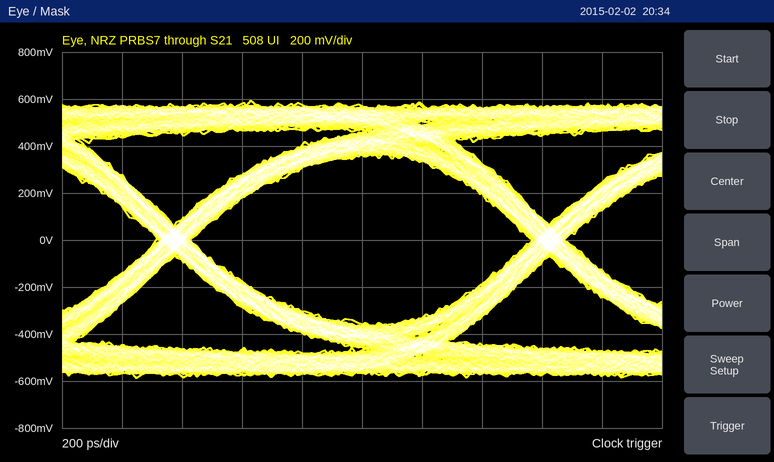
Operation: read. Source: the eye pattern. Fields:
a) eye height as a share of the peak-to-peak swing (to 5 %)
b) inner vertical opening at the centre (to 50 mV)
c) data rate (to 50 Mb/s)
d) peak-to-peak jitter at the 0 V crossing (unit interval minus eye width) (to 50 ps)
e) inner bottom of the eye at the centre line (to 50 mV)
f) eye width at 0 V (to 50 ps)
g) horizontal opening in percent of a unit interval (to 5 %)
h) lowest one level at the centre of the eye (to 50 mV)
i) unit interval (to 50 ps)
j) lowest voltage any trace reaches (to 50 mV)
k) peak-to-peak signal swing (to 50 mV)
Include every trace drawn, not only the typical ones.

60 %
700 mV
800 Mb/s
100 ps
-350 mV
1.15 ns
90 %
350 mV
1.25 ns
-600 mV
1.20 V
